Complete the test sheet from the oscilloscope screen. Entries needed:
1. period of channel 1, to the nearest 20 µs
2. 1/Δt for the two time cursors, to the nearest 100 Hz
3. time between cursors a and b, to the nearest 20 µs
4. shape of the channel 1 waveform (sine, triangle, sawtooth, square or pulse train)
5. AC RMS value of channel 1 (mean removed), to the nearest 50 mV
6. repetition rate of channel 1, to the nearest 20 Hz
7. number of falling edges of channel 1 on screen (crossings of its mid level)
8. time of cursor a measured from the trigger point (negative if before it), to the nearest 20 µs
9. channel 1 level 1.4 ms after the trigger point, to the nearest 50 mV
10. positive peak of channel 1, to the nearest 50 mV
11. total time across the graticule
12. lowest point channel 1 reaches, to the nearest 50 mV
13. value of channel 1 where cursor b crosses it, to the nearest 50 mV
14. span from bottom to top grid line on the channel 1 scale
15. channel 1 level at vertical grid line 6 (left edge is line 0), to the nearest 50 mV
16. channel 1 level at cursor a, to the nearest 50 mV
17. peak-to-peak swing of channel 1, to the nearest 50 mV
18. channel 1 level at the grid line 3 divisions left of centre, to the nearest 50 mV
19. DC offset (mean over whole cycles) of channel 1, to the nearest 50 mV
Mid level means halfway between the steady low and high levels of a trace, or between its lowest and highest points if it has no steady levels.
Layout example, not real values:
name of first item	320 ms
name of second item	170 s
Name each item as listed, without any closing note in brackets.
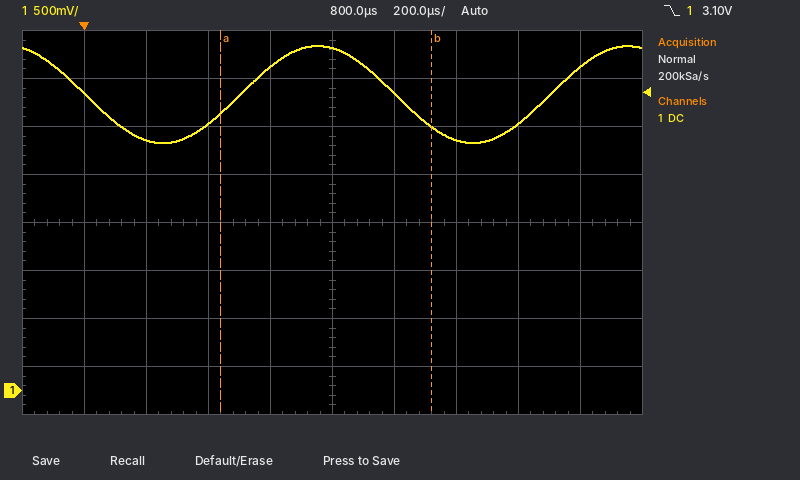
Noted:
period of channel 1, to the nearest 20 µs	1.00 ms
1/Δt for the two time cursors, to the nearest 100 Hz	1.5 kHz
time between cursors a and b, to the nearest 20 µs	680 µs
shape of the channel 1 waveform	sine
AC RMS value of channel 1 (mean removed), to the nearest 50 mV	350 mV
repetition rate of channel 1, to the nearest 20 Hz	1.00 kHz
number of falling edges of channel 1 on screen	2
time of cursor a measured from the trigger point (negative if before it), to the nearest 20 µs	+440 µs
channel 1 level 1.4 ms after the trigger point, to the nearest 50 mV	2.80 V
positive peak of channel 1, to the nearest 50 mV	3.60 V
total time across the graticule	2 ms
lowest point channel 1 reaches, to the nearest 50 mV	2.60 V
value of channel 1 where cursor b crosses it, to the nearest 50 mV	2.75 V
span from bottom to top grid line on the channel 1 scale	4 V
channel 1 level at vertical grid line 6 (left edge is line 0), to the nearest 50 mV	3.10 V
channel 1 level at cursor a, to the nearest 50 mV	2.90 V
peak-to-peak swing of channel 1, to the nearest 50 mV	1.00 V
channel 1 level at the grid line 3 divisions left of centre, to the nearest 50 mV	2.60 V
DC offset (mean over whole cycles) of channel 1, to the nearest 50 mV	3.10 V
